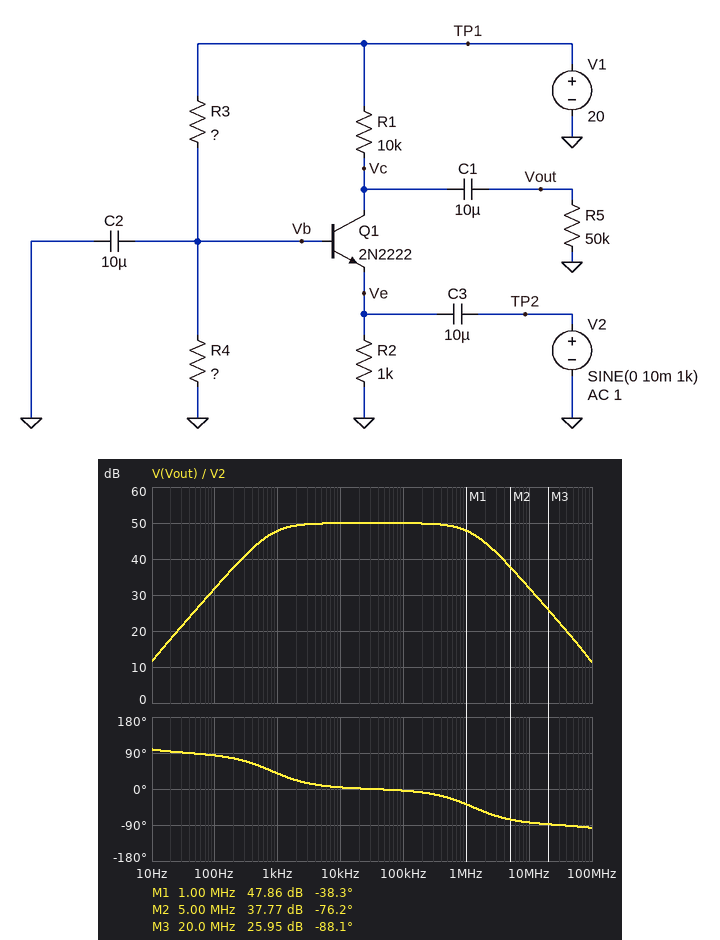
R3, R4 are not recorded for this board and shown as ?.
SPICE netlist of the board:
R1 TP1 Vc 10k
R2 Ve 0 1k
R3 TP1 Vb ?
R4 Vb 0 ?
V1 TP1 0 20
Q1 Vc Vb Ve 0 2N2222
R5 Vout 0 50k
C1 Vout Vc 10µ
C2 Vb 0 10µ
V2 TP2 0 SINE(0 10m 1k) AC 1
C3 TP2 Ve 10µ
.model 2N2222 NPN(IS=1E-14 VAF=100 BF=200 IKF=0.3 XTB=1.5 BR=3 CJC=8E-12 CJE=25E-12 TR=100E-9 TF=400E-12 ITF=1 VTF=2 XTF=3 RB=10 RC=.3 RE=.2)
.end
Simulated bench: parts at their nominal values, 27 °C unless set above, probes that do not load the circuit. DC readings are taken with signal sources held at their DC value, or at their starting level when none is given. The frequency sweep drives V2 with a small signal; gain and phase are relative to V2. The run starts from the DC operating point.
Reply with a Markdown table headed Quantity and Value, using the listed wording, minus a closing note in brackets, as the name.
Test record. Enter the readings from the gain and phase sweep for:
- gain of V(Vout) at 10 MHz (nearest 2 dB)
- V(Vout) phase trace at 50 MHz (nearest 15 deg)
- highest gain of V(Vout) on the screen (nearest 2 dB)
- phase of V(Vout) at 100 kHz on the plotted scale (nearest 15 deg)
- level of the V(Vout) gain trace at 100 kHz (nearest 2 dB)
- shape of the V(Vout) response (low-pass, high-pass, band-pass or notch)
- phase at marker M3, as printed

| Quantity | Value |
|---|---|
| gain of V(Vout) at 10 MHz | 32 dB |
| V(Vout) phase trace at 50 MHz | -90 deg |
| highest gain of V(Vout) on the screen | 50 dB |
| phase of V(Vout) at 100 kHz on the plotted scale | 0 deg |
| level of the V(Vout) gain trace at 100 kHz | 50 dB |
| shape of the V(Vout) response | band-pass |
| phase at marker M3, as printed | -88.1 deg |
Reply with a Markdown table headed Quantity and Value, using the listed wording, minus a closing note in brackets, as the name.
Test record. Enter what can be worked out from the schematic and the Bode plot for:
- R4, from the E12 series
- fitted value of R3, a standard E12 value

| Quantity | Value |
|---|---|
| R4, from the E12 series | 10 kΩ |
| fitted value of R3, a standard E12 value | 68 kΩ |
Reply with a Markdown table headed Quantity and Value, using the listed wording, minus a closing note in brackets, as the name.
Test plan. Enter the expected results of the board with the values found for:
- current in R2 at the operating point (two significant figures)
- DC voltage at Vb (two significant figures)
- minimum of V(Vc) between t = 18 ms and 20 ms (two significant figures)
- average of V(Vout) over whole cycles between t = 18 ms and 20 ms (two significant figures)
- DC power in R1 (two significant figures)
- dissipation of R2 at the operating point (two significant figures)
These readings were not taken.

| Quantity | Value |
|---|---|
| current in R2 at the operating point | 1.8 mA |
| DC voltage at Vb | 2.5 V |
| minimum of V(Vc) between t = 18 ms and 20 ms | 1.8 V |
| average of V(Vout) over whole cycles between t = 18 ms and 20 ms | 1.1 V |
| DC power in R1 | 32 mW |
| dissipation of R2 at the operating point | 3.3 mW |
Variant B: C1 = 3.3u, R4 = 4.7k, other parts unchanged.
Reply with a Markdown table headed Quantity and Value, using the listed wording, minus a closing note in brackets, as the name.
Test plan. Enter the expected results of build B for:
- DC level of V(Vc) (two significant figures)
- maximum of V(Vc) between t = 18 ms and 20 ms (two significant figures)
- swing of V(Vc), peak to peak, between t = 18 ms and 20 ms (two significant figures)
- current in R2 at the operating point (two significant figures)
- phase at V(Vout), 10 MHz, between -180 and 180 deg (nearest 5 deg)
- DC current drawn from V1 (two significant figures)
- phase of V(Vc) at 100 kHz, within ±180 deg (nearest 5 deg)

| Quantity | Value |
|---|---|
| DC level of V(Vc) | 14 V |
| maximum of V(Vc) between t = 18 ms and 20 ms | 15 V |
| swing of V(Vc), peak to peak, between t = 18 ms and 20 ms | 3.6 V |
| current in R2 at the operating point | 640 µA |
| phase at V(Vout), 10 MHz, between -180 and 180 deg | -65 deg |
| DC current drawn from V1 | 910 µA |
| phase of V(Vc) at 100 kHz, within ±180 deg | 0 deg |
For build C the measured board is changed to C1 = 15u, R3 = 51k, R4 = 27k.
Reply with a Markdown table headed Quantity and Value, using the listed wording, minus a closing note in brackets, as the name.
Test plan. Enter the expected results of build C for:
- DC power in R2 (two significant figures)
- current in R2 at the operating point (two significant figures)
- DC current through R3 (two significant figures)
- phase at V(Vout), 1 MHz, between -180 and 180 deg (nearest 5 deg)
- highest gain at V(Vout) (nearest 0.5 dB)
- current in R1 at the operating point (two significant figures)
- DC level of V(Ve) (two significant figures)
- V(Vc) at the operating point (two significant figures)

| Quantity | Value |
|---|---|
| DC power in R2 | 4.1 mW |
| current in R2 at the operating point | 2.0 mA |
| DC current through R3 | 340 µA |
| phase at V(Vout), 1 MHz, between -180 and 180 deg | -30 deg |
| highest gain at V(Vout) | 8.0 dB |
| current in R1 at the operating point | 1.8 mA |
| DC level of V(Ve) | 2.0 V |
| V(Vc) at the operating point | 2.1 V |
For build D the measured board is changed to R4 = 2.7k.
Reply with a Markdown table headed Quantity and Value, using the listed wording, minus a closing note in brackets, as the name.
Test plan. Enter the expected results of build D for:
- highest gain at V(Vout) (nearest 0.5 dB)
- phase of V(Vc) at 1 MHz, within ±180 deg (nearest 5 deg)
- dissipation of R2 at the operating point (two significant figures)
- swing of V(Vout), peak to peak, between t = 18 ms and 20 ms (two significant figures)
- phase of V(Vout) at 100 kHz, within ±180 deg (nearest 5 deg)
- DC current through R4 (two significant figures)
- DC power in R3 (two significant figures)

| Quantity | Value |
|---|---|
| highest gain at V(Vout) | 34.0 dB |
| phase of V(Vc) at 1 MHz, within ±180 deg | -10 deg |
| dissipation of R2 at the operating point | 25 µW |
| swing of V(Vout), peak to peak, between t = 18 ms and 20 ms | 990 mV |
| phase of V(Vout) at 100 kHz, within ±180 deg | 0 deg |
| DC current through R4 | 280 µA |
| DC power in R3 | 5.4 mW |
